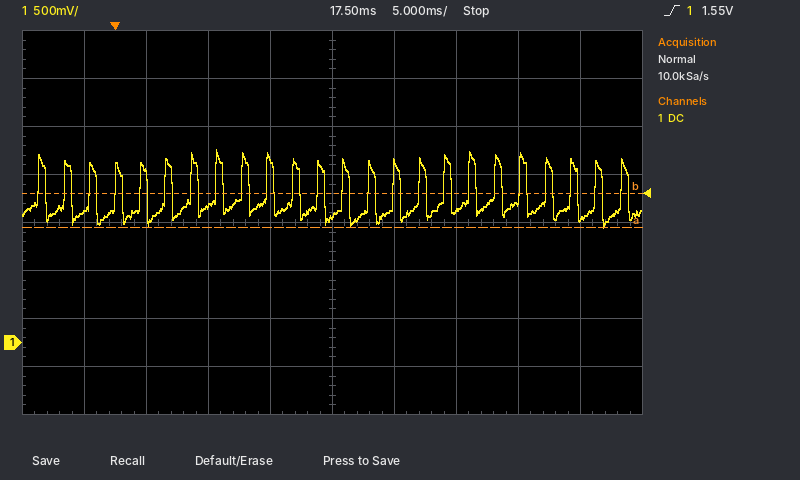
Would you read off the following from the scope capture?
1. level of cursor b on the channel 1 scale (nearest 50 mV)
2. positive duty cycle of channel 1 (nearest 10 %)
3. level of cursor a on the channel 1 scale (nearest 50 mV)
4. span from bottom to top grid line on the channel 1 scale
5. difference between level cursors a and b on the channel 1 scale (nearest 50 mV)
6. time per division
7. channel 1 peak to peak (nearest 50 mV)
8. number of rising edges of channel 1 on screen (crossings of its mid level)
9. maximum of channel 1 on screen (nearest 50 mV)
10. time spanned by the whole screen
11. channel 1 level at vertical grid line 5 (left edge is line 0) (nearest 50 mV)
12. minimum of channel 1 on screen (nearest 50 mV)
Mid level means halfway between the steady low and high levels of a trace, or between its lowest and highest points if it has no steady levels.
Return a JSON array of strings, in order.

["1.55 V", "30 %", "1.20 V", "4 V", "350 mV", "5 ms", "800 mV", "24", "2.00 V", "50 ms", "1.30 V", "1.20 V"]
